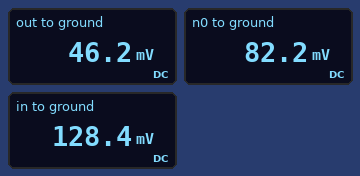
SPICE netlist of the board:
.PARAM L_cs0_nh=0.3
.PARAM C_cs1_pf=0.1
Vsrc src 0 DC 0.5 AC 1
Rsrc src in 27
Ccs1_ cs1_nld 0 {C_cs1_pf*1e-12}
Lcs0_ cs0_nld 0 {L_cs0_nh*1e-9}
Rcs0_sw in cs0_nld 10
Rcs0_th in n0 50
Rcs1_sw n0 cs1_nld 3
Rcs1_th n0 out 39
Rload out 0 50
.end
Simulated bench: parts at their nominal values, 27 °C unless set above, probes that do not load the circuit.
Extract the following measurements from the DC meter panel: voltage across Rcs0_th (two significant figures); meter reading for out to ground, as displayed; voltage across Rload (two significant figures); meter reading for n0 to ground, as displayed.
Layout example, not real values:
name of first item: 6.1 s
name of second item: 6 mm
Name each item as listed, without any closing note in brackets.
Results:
voltage across Rcs0_th: 46 mV
meter reading for out to ground, as displayed: 46.2 mV
voltage across Rload: 46 mV
meter reading for n0 to ground, as displayed: 82.2 mV
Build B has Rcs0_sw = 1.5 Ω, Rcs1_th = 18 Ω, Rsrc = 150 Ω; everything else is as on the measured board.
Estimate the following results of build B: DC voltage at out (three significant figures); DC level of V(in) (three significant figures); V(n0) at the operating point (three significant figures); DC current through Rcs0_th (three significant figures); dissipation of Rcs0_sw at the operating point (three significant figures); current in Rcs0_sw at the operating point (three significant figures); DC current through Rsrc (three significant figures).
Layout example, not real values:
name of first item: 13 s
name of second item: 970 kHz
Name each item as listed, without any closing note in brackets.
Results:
DC voltage at out: 2.07 mV
DC level of V(in): 4.89 mV
V(n0) at the operating point: 2.82 mV
DC current through Rcs0_th: 41.4 µA
dissipation of Rcs0_sw at the operating point: 15.9 µW
current in Rcs0_sw at the operating point: 3.26 mA
DC current through Rsrc: 3.30 mA
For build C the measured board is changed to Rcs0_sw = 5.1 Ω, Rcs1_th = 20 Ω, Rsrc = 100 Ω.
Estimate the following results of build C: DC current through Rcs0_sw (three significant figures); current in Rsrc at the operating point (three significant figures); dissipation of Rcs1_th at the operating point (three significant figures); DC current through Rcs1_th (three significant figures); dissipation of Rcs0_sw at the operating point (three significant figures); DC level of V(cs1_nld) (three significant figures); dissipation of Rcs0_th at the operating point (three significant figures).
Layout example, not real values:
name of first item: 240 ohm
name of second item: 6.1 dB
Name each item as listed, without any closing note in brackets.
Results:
DC current through Rcs0_sw: 4.57 mA
current in Rsrc at the operating point: 4.77 mA
dissipation of Rcs1_th at the operating point: 755 nW
DC current through Rcs1_th: 194 µA
dissipation of Rcs0_sw at the operating point: 107 µW
DC level of V(cs1_nld): 13.6 mV
dissipation of Rcs0_th at the operating point: 1.89 µW
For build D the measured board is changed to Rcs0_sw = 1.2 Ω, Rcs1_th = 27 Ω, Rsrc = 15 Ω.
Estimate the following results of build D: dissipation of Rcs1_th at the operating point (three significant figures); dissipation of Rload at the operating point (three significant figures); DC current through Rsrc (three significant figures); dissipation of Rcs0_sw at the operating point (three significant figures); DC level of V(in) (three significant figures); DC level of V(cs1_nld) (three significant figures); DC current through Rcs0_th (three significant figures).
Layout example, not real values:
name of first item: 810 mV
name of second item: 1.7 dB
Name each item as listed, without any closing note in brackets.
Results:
dissipation of Rcs1_th at the operating point: 2.26 µW
dissipation of Rload at the operating point: 4.18 µW
DC current through Rsrc: 30.9 mA
dissipation of Rcs0_sw at the operating point: 1.12 mW
DC level of V(in): 36.7 mV
DC level of V(cs1_nld): 22.3 mV
DC current through Rcs0_th: 289 µA
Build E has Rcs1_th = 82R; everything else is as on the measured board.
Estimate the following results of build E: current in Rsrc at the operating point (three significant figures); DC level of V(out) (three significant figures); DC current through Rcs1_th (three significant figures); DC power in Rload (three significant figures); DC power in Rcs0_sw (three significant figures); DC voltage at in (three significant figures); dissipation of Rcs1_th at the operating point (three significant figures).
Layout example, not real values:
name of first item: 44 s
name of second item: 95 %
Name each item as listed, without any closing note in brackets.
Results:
current in Rsrc at the operating point: 13.7 mA
DC level of V(out): 35.7 mV
DC current through Rcs1_th: 714 µA
DC power in Rload: 25.5 µW
DC power in Rcs0_sw: 1.69 mW
DC voltage at in: 130 mV
dissipation of Rcs1_th at the operating point: 41.8 µW
